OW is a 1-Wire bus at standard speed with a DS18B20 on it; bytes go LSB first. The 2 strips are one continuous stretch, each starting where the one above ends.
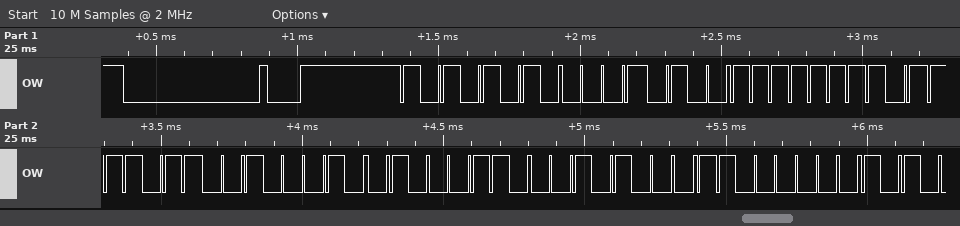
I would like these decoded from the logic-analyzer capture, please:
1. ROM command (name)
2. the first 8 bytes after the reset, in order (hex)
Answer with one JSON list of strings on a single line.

["Match ROM", "55 28 FF DE 44 62 14 03"]
